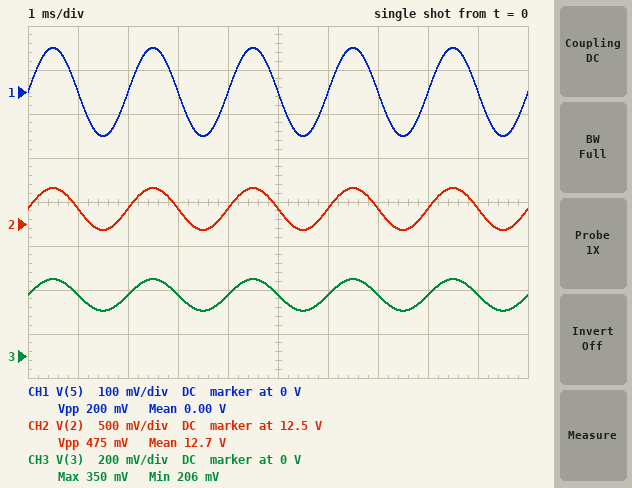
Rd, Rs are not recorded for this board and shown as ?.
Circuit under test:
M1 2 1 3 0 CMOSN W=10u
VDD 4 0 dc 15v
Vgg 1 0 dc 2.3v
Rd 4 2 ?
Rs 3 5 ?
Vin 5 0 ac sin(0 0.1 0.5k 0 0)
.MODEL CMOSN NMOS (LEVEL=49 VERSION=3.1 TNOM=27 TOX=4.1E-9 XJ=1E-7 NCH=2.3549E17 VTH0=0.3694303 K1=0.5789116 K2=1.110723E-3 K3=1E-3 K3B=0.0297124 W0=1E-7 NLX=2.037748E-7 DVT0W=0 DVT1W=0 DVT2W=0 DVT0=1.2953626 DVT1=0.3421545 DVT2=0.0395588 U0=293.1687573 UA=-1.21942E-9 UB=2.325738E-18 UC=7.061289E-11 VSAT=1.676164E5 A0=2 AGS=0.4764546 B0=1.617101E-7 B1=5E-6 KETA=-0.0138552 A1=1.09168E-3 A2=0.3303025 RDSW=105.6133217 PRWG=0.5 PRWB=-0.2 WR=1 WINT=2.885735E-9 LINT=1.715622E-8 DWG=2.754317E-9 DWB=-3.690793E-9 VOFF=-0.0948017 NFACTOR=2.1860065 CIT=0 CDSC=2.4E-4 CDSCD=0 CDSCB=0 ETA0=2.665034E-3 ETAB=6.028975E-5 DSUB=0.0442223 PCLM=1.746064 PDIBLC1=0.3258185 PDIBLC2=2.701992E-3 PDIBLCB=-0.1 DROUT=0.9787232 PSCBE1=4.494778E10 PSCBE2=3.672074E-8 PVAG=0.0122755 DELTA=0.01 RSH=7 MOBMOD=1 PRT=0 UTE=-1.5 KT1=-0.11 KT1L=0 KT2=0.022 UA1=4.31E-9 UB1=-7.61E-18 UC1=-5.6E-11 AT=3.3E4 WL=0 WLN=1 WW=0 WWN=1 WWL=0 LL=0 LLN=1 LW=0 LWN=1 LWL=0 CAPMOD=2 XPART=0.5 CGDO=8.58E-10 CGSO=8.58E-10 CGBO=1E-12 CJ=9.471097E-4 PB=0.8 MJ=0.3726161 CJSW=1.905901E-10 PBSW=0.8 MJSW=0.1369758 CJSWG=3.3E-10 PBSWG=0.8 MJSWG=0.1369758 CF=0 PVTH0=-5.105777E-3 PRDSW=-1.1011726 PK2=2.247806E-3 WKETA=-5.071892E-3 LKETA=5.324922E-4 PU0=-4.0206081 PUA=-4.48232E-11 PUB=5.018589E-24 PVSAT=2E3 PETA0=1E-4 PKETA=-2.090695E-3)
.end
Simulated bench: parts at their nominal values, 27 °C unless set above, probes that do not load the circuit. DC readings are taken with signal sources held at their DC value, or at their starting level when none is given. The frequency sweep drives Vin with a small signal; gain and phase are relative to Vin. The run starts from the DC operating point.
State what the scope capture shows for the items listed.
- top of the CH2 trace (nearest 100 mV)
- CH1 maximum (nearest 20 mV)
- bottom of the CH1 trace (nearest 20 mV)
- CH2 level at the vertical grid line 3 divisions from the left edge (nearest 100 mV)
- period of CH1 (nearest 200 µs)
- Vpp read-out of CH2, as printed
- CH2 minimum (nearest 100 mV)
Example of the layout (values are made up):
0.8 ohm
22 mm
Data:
12.9 V
100 mV
-100 mV
12.7 V
2.0 ms
475 mV
12.4 V
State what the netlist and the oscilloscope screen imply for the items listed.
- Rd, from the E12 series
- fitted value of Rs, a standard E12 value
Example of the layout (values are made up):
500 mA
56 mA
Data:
4.7 kΩ
560 Ω
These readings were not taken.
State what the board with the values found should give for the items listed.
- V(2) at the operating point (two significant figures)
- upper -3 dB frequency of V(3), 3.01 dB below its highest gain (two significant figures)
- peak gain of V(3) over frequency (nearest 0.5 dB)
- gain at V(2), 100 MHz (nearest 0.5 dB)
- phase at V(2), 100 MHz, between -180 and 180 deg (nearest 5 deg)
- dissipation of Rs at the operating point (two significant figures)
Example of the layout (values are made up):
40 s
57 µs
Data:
13 V
2.1 GHz
-3.0 dB
7.5 dB
-15 deg
140 µW
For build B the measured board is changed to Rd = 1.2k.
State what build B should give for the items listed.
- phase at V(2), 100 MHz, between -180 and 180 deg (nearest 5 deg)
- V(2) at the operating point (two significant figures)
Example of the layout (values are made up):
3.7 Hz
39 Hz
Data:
-10 deg
14 V
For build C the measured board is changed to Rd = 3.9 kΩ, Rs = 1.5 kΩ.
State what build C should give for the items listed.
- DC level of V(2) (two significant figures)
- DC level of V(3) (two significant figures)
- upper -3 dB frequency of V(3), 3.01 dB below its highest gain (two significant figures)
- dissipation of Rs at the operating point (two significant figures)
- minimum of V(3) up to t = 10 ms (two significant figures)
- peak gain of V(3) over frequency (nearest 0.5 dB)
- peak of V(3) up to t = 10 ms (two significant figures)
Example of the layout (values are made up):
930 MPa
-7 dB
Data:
14 V
510 mV
1.1 GHz
180 µW
460 mV
-5.5 dB
570 mV
